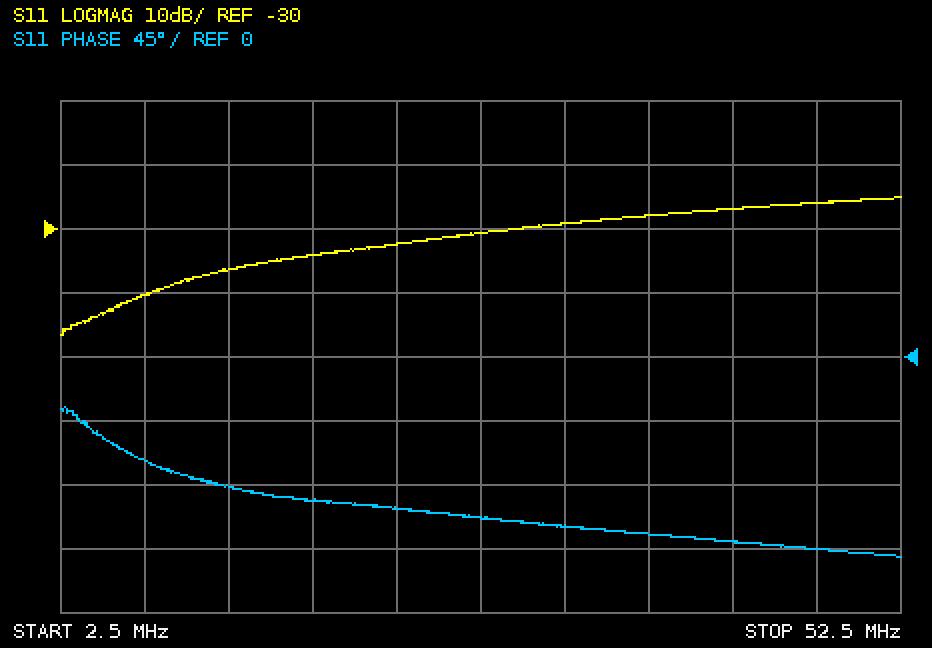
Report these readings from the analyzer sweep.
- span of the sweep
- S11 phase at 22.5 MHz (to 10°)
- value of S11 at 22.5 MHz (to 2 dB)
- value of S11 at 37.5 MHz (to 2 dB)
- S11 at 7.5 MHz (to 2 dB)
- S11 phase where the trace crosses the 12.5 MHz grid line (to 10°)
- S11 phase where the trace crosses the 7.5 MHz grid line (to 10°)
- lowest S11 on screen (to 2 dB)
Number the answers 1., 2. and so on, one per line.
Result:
1. 50 MHz
2. -110°
3. -32 dB
4. -28 dB
5. -40 dB
6. -90°
7. -70°
8. -46 dB
